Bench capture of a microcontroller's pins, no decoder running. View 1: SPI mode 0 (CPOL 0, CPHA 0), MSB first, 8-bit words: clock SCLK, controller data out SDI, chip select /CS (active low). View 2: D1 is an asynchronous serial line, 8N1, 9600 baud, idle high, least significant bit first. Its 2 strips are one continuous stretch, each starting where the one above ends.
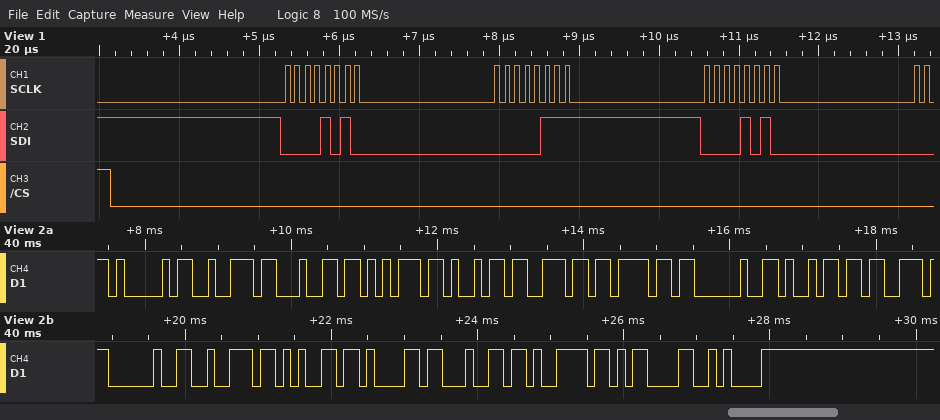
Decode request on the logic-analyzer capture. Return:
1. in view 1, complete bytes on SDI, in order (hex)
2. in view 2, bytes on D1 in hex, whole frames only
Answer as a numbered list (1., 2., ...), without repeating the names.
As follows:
1. 0A 07 0A
2. 0x41 0x72 0x64 0x75 0x69 0x6E 0x6F 0x20 0x69 0x73 0x20 0x72 0x65 0x61 0x64 0x79 0x0D 0x0A
